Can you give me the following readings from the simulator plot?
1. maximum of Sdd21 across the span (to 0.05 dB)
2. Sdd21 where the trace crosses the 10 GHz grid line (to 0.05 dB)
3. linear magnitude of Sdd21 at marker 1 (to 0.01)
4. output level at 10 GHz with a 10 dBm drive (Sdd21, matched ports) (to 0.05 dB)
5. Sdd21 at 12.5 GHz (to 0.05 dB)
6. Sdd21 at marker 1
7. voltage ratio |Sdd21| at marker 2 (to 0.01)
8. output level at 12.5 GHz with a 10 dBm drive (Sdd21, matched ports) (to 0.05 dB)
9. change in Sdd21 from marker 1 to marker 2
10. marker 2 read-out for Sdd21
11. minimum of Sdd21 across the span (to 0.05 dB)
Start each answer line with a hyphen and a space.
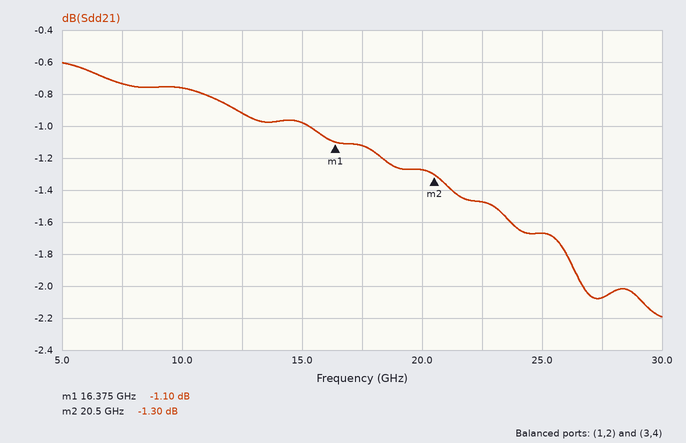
- -0.60 dB
- -0.75 dB
- 0.88
- 9.25 dBm
- -0.90 dB
- -1.10 dB
- 0.86
- 9.10 dBm
- -0.20 dB
- -1.30 dB
- -2.20 dB
